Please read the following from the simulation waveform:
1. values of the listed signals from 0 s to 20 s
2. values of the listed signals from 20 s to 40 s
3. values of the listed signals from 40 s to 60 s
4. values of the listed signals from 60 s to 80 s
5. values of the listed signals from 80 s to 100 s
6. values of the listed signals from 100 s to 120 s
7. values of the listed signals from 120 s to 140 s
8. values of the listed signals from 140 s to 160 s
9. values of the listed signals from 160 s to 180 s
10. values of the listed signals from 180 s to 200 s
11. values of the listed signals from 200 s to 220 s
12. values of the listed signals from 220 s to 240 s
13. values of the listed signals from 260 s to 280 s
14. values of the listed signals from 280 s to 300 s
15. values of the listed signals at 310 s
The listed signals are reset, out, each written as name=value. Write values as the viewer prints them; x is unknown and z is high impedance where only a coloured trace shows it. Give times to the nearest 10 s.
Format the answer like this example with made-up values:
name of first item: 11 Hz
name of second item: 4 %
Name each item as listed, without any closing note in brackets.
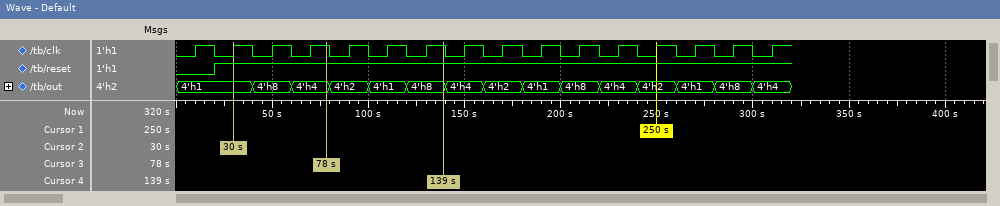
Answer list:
values of the listed signals from 0 s to 20 s: reset=0, out=4'h1
values of the listed signals from 20 s to 40 s: reset=1, out=4'h1
values of the listed signals from 40 s to 60 s: reset=1, out=4'h8
values of the listed signals from 60 s to 80 s: reset=1, out=4'h4
values of the listed signals from 80 s to 100 s: reset=1, out=4'h2
values of the listed signals from 100 s to 120 s: reset=1, out=4'h1
values of the listed signals from 120 s to 140 s: reset=1, out=4'h8
values of the listed signals from 140 s to 160 s: reset=1, out=4'h4
values of the listed signals from 160 s to 180 s: reset=1, out=4'h2
values of the listed signals from 180 s to 200 s: reset=1, out=4'h1
values of the listed signals from 200 s to 220 s: reset=1, out=4'h8
values of the listed signals from 220 s to 240 s: reset=1, out=4'h4
values of the listed signals from 260 s to 280 s: reset=1, out=4'h1
values of the listed signals from 280 s to 300 s: reset=1, out=4'h8
values of the listed signals at 310 s: reset=1, out=4'h4
